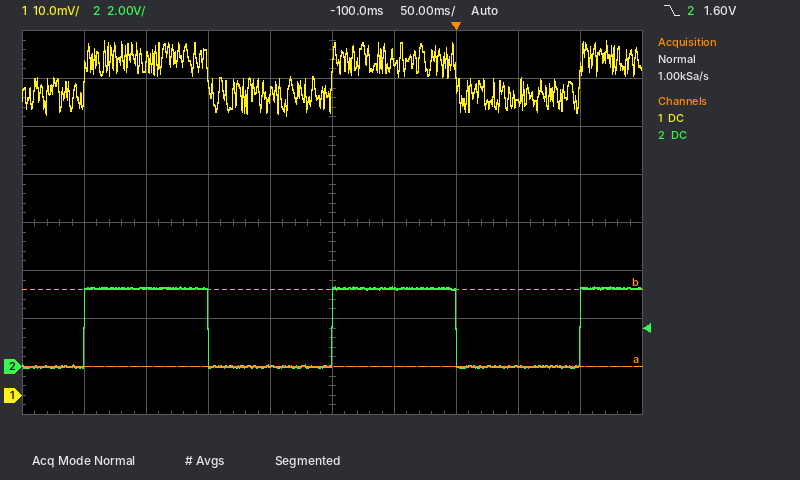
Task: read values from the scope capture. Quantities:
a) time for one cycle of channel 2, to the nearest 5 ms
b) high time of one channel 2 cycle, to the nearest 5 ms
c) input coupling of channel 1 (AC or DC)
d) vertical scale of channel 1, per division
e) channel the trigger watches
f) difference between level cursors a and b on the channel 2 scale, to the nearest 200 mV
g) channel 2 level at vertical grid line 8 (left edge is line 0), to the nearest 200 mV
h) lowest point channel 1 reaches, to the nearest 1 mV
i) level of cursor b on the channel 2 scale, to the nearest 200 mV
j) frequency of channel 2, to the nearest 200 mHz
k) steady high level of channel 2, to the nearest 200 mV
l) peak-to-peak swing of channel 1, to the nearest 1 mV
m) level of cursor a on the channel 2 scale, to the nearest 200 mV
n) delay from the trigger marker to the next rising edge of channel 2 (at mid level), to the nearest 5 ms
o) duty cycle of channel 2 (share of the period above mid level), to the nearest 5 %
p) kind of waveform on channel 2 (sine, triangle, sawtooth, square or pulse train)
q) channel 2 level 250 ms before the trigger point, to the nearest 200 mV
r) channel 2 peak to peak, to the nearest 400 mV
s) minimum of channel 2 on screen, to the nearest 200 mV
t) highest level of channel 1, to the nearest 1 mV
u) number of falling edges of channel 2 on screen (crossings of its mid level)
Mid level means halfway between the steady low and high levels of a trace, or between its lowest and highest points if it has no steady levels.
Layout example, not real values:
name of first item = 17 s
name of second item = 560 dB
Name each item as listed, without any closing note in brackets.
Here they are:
time for one cycle of channel 2, to the nearest 5 ms = 200 ms
high time of one channel 2 cycle, to the nearest 5 ms = 100 ms
input coupling of channel 1 = DC
vertical scale of channel 1, per division = 10 mV
channel the trigger watches = channel 2
difference between level cursors a and b on the channel 2 scale, to the nearest 200 mV = 3.2 V
channel 2 level at vertical grid line 8 (left edge is line 0), to the nearest 200 mV = 0.0 V
lowest point channel 1 reaches, to the nearest 1 mV = 58 mV
level of cursor b on the channel 2 scale, to the nearest 200 mV = 3.2 V
frequency of channel 2, to the nearest 200 mHz = 5.0 Hz
steady high level of channel 2, to the nearest 200 mV = 3.2 V
peak-to-peak swing of channel 1, to the nearest 1 mV = 16 mV
level of cursor a on the channel 2 scale, to the nearest 200 mV = 0.0 V
delay from the trigger marker to the next rising edge of channel 2 (at mid level), to the nearest 5 ms = 100 ms
duty cycle of channel 2 (share of the period above mid level), to the nearest 5 % = 50 %
kind of waveform on channel 2 = square
channel 2 level 250 ms before the trigger point, to the nearest 200 mV = 3.2 V
channel 2 peak to peak, to the nearest 400 mV = 3.2 V
minimum of channel 2 on screen, to the nearest 200 mV = 0.0 V
highest level of channel 1, to the nearest 1 mV = 74 mV
number of falling edges of channel 2 on screen = 2
